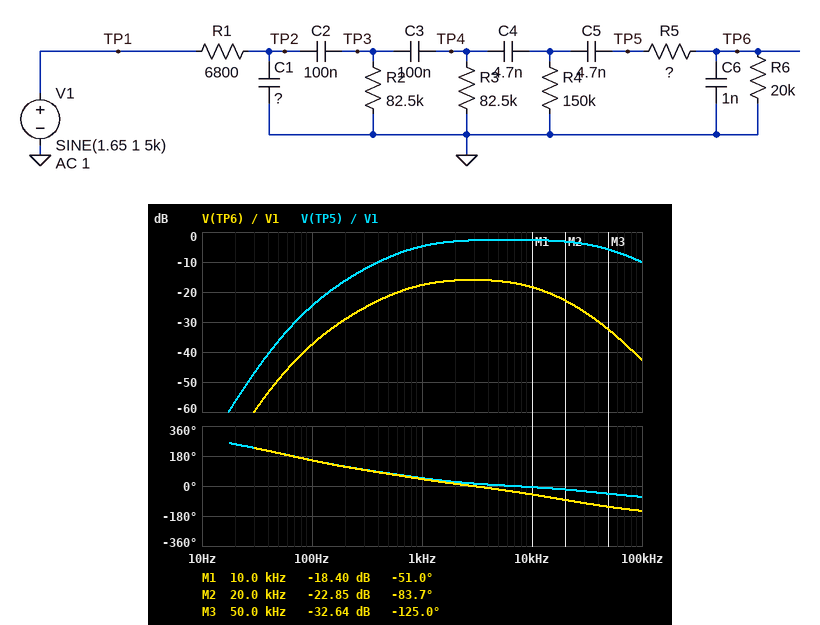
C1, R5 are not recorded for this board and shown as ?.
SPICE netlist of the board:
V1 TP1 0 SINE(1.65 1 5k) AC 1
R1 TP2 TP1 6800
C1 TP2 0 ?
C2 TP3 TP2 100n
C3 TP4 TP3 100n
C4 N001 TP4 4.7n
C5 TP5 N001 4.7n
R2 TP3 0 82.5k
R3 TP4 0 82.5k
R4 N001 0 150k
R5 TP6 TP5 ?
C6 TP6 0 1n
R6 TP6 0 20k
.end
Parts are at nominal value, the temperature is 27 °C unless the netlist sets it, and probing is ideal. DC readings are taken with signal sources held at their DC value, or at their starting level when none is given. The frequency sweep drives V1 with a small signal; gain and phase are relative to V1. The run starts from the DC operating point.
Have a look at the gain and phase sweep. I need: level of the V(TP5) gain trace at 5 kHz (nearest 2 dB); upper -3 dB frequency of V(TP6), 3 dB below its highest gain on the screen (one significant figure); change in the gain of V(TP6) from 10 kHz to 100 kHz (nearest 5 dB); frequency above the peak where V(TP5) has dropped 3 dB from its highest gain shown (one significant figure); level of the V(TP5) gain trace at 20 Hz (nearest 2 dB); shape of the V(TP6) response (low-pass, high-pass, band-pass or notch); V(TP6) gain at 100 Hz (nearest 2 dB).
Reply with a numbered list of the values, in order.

1. -2 dB
2. 10 kHz
3. -25 dB
4. 50 kHz
5. -56 dB
6. band-pass
7. -38 dB
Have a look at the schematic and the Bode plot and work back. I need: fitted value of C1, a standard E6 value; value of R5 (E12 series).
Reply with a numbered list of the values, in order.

1. 680 pF
2. 68 kΩ
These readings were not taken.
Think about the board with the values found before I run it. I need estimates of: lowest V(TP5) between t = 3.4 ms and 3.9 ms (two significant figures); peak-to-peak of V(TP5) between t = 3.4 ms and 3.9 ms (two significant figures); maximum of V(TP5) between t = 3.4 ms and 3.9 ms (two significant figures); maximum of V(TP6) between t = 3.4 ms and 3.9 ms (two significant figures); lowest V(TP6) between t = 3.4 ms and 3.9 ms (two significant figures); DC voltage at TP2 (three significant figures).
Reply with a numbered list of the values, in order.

1. -740 mV
2. 1.5 V
3. 740 mV
4. 150 mV
5. -150 mV
6. 1.65 V
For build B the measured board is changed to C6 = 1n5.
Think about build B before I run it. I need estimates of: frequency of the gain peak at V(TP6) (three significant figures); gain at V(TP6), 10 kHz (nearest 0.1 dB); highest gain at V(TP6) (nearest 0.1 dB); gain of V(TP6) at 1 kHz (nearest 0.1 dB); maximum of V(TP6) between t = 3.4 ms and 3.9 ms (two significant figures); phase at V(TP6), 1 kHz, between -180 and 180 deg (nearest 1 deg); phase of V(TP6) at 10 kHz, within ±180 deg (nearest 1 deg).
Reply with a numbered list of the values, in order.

1. 2.40 kHz
2. -20.5 dB
3. -16.4 dB
4. -17.8 dB
5. 140 mV
6. 39 deg
7. -62 deg
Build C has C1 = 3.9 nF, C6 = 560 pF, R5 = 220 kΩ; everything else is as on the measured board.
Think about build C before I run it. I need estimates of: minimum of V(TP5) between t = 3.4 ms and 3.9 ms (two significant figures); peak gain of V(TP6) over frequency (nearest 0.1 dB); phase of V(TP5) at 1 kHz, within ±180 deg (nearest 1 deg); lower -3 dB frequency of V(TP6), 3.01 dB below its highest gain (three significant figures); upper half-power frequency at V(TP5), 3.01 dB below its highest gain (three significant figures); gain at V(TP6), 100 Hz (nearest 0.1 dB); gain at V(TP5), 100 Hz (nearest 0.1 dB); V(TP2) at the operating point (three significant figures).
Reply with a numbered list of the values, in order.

1. -660 mV
2. -24.1 dB
3. 23 deg
4. 402 Hz
5. 8.31 kHz
6. -39.1 dB
7. -17.5 dB
8. 1.65 V
